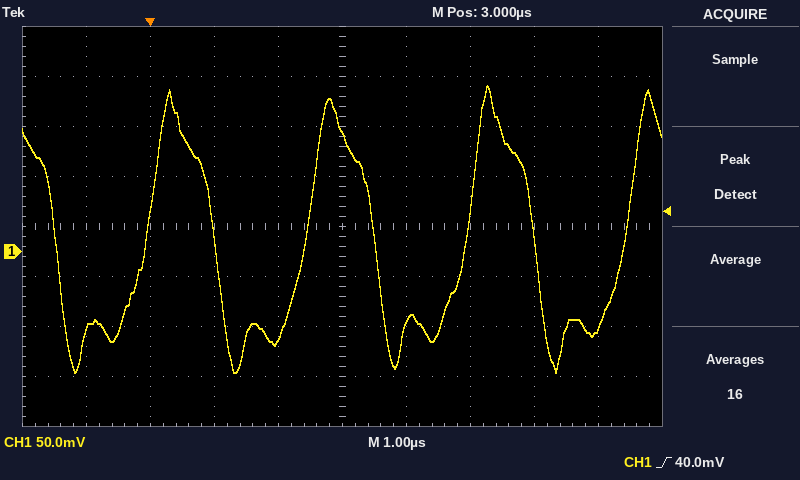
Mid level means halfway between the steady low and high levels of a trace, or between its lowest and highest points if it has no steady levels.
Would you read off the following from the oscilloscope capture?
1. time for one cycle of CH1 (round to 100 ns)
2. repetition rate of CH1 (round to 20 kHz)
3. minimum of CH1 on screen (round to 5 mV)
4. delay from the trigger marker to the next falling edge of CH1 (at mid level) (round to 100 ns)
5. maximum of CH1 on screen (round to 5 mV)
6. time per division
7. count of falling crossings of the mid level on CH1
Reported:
2.5 µs
400 kHz
-120 mV
1.0 µs
165 mV
1 µs
4
